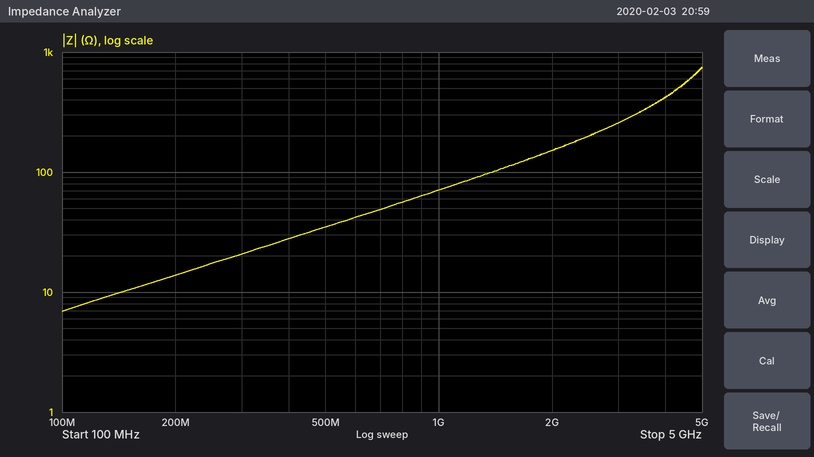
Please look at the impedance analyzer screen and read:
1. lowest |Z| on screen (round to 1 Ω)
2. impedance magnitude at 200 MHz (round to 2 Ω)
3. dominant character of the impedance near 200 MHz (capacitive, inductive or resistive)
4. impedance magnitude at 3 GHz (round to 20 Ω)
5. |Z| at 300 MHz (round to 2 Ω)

7 Ω
14 Ω
inductive
260 Ω
20 Ω
